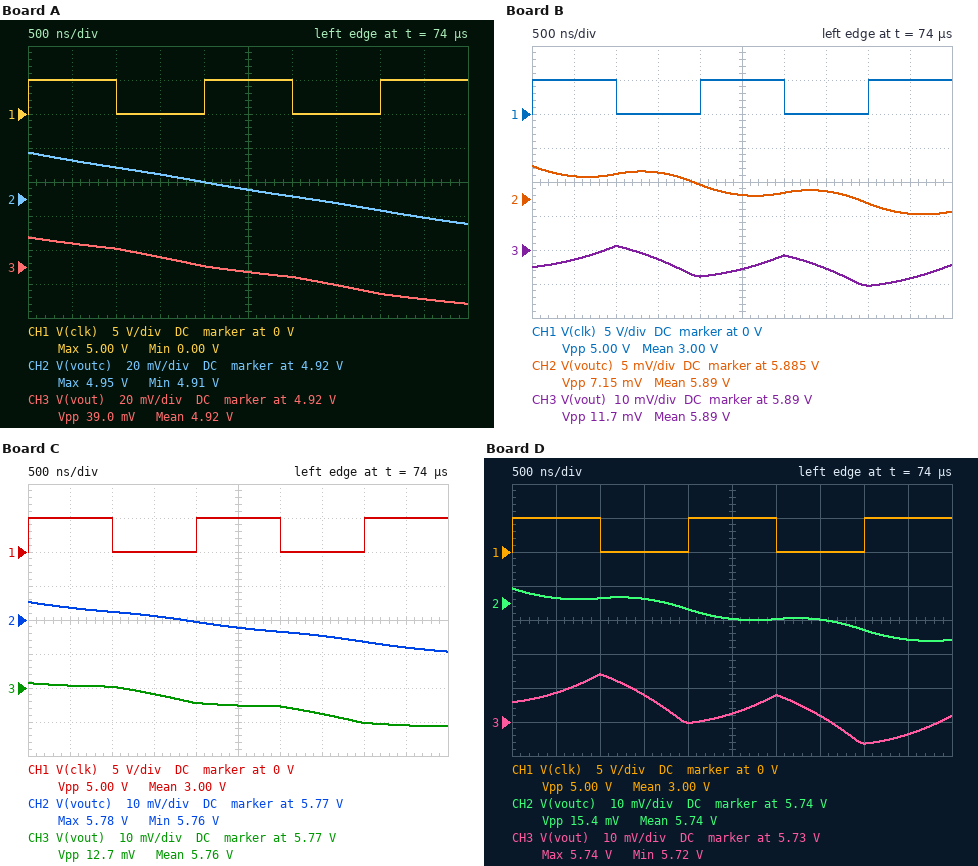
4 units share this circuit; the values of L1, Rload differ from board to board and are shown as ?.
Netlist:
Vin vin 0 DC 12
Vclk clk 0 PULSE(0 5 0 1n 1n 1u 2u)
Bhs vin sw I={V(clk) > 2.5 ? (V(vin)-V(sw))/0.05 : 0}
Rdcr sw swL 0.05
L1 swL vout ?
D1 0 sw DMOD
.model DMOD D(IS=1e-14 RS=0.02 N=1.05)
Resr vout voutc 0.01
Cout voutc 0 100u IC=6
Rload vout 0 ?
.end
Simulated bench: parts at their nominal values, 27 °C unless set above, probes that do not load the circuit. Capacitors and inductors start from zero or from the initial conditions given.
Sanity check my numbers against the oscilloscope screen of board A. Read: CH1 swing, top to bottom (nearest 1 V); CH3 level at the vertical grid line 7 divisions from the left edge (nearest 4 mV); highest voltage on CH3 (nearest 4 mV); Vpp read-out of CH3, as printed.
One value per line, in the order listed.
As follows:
5 V
4.908 V
4.936 V
39.0 mV
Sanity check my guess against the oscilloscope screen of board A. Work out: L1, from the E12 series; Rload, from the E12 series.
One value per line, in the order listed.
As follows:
33 µH
3.3 Ω
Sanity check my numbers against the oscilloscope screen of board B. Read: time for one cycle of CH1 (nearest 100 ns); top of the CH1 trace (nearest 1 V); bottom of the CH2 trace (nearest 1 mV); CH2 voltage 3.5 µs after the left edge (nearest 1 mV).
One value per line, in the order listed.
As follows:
2.0 µs
5 V
5.883 V
5.886 V
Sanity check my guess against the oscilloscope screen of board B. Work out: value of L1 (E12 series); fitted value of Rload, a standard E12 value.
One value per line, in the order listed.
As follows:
8.2 µH
12 Ω
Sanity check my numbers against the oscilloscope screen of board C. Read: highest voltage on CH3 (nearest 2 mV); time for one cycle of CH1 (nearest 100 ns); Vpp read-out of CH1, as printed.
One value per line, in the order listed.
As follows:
5.772 V
2.0 µs
5.00 V
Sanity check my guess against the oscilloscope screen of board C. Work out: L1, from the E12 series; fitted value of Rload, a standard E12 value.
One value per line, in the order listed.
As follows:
33 µH
15 Ω
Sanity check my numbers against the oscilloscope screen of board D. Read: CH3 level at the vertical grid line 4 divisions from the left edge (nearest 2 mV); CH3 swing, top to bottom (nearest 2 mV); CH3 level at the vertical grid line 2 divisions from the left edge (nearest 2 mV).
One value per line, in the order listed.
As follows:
5.730 V
20 mV
5.744 V
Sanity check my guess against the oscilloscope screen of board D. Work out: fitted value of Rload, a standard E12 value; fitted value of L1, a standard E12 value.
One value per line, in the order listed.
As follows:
6.8 Ω
5.6 µH
